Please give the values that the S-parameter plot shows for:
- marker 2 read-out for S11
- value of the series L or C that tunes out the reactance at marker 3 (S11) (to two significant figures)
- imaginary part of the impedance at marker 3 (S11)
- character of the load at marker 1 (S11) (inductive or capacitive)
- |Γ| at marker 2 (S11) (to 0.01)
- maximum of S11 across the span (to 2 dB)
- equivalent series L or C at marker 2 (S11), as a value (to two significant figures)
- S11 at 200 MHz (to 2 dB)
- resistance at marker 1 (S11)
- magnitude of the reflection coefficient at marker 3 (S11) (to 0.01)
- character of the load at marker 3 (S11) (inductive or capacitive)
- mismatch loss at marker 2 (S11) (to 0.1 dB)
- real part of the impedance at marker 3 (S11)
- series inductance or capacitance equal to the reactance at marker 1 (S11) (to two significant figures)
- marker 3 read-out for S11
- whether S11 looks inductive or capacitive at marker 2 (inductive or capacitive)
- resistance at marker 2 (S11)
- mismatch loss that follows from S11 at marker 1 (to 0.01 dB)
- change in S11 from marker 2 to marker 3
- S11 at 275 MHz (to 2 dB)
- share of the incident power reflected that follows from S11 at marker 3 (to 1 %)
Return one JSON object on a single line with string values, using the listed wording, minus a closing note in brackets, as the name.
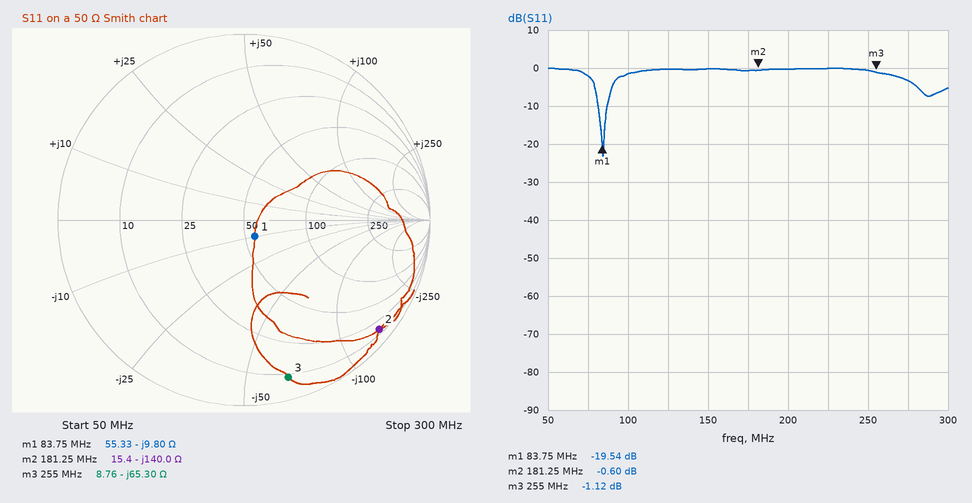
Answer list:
{"marker 2 read-out for S11": "-0.60 dB", "value of the series L or C that tunes out the reactance at marker 3 (S11)": "41 nH", "imaginary part of the impedance at marker 3": "-65.30 Ω", "character of the load at marker 1 (S11)": "capacitive", "|Γ| at marker 2 (S11)": "0.93", "maximum of S11 across the span": "0 dB", "equivalent series L or C at marker 2 (S11), as a value": "6.3 pF", "S11 at 200 MHz": "0 dB", "resistance at marker 1": "55.33 Ω", "magnitude of the reflection coefficient at marker 3 (S11)": "0.88", "character of the load at marker 3 (S11)": "capacitive", "mismatch loss at marker 2 (S11)": "8.9 dB", "real part of the impedance at marker 3": "8.76 Ω", "series inductance or capacitance equal to the reactance at marker 1 (S11)": "190 pF", "marker 3 read-out for S11": "-1.12 dB", "whether S11 looks inductive or capacitive at marker 2": "capacitive", "resistance at marker 2": "15.4 Ω", "mismatch loss that follows from S11 at marker 1": "0.05 dB", "change in S11 from marker 2 to marker 3": "-0.52 dB", "S11 at 275 MHz": "-4 dB", "share of the incident power reflected that follows from S11 at marker 3": "77 %"}
